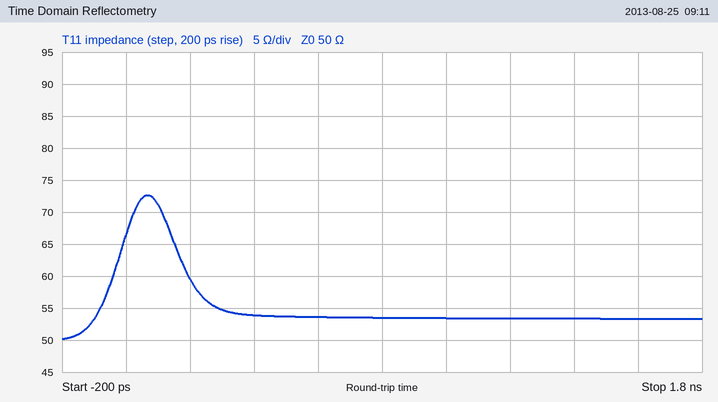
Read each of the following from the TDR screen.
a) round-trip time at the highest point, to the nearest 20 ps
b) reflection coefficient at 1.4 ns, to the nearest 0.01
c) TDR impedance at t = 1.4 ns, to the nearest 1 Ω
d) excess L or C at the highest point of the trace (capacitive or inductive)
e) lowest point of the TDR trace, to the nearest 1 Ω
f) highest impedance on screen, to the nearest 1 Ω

60 ps
+0.03
53 Ω
inductive
50 Ω
73 Ω
